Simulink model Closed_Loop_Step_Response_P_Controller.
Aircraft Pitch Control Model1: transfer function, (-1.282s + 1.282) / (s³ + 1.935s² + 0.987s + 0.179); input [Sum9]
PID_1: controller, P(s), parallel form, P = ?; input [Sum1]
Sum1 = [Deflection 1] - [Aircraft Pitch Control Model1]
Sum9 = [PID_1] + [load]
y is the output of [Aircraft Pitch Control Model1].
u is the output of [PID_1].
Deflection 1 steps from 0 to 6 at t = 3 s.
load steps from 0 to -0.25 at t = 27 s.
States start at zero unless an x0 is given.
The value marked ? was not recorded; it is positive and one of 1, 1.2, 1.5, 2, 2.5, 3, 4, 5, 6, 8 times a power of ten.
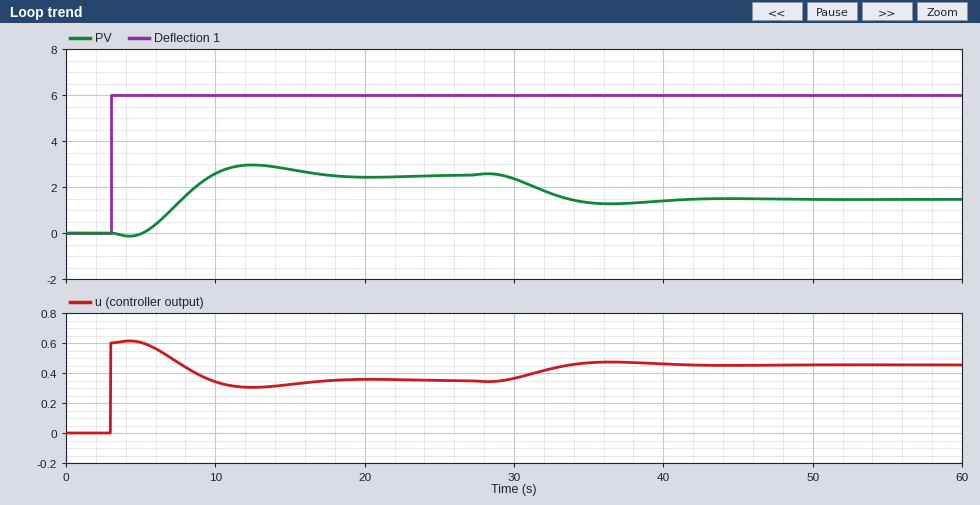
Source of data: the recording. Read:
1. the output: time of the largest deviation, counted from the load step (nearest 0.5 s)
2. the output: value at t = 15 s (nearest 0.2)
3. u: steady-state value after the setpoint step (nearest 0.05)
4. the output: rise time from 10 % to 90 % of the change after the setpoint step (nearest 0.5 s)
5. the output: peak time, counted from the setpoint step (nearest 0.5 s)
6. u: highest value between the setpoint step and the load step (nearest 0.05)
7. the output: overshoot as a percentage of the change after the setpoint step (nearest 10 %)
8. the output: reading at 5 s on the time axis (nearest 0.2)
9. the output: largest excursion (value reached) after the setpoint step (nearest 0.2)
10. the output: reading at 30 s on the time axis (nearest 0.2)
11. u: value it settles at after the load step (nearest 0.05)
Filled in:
9.5 s
2.8
0.35
3.5 s
9.5 s
0.60
20 %
0.0
3.0
2.4
0.45
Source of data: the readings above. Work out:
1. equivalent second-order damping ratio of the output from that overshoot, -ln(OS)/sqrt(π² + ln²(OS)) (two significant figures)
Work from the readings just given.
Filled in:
0.46
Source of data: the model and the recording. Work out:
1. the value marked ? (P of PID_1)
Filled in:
0.1
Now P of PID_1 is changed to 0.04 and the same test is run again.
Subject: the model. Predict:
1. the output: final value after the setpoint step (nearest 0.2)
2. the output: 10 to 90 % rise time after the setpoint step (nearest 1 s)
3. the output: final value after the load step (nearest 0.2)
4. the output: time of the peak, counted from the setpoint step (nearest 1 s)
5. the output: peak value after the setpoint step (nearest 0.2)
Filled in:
1.4
5 s
0.0
12 s
1.4
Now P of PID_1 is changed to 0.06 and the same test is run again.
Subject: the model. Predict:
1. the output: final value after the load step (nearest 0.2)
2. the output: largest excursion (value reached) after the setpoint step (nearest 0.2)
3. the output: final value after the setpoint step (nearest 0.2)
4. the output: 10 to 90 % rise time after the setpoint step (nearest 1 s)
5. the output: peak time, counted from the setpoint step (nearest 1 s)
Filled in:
0.6
2.0
1.8
4 s
11 s
